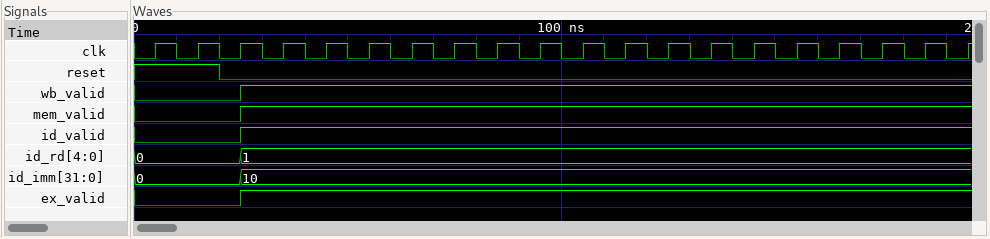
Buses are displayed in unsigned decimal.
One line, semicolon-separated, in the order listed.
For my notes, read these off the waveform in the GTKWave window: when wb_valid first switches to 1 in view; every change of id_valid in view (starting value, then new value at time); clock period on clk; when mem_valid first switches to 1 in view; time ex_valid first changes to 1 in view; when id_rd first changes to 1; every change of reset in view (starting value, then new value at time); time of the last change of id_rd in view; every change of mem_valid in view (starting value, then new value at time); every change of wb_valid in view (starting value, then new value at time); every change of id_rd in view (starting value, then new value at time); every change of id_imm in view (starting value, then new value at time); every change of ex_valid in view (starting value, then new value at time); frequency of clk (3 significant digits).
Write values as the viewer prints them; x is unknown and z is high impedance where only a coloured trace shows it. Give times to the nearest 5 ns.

25 ns; 0, 1 at 25 ns; 10 ns; 25 ns; 25 ns; 25 ns; 1, 0 at 20 ns; 25 ns; 0, 1 at 25 ns; 0, 1 at 25 ns; 0, 1 at 25 ns; 0, 10 at 25 ns; 0, 1 at 25 ns; 100 MHz
